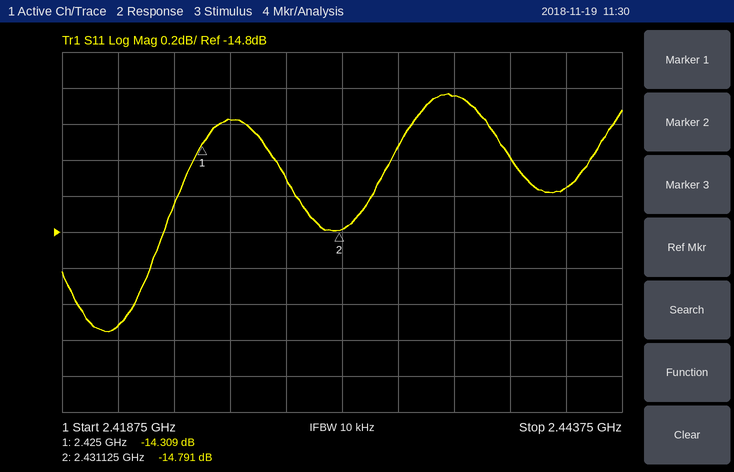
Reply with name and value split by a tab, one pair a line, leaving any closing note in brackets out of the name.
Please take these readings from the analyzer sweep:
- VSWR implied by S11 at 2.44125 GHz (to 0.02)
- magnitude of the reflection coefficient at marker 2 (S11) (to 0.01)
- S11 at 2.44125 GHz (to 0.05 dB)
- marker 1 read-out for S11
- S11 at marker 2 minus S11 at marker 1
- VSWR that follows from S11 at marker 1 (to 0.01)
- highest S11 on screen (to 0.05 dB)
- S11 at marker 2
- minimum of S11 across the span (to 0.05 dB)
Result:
VSWR implied by S11 at 2.44125 GHz	1.46
magnitude of the reflection coefficient at marker 2 (S11)	0.18
S11 at 2.44125 GHz	-14.55 dB
marker 1 read-out for S11	-14.309 dB
S11 at marker 2 minus S11 at marker 1	-0.482 dB
VSWR that follows from S11 at marker 1	1.48
highest S11 on screen	-14.05 dB
S11 at marker 2	-14.791 dB
minimum of S11 across the span	-15.35 dB
